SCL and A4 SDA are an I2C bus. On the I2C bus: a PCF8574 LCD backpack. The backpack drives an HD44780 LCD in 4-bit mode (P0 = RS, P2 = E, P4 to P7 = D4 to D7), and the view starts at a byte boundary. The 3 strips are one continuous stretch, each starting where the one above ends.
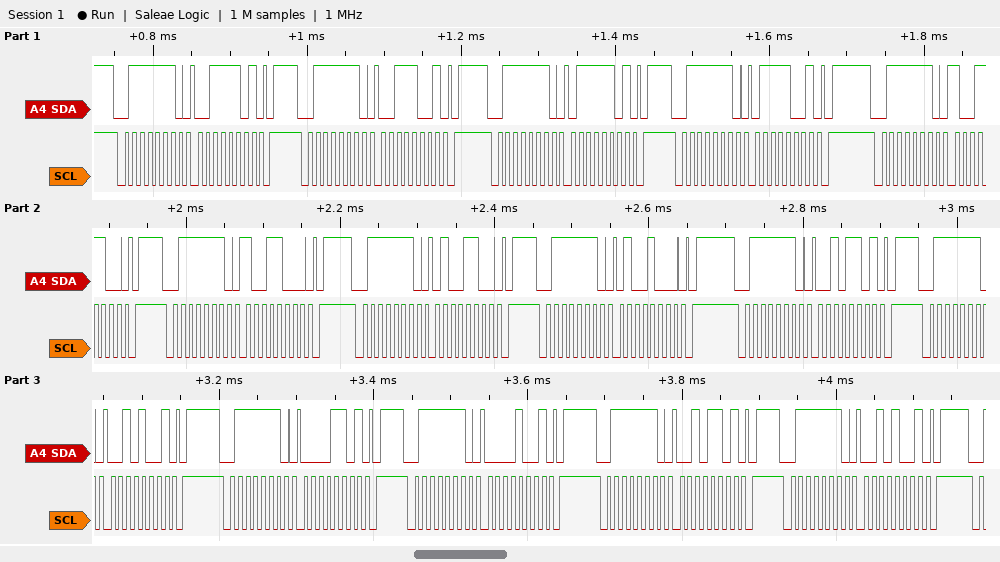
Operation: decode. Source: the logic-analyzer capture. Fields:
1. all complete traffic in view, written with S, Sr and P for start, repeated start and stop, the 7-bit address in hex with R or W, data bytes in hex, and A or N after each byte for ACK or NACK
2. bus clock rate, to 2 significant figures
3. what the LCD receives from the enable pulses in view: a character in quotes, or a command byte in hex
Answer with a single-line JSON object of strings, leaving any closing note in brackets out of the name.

{"all complete traffic in view, written with S, Sr and P for start, repeated start and stop, the 7-bit address in hex with R or W, data bytes in hex, and A or N after each byte for ACK or NACK": "S 3FW A 3D A P S 3FW A 39 A P S 3FW A 7D A P S 3FW A 79 A P S 3FW A 9C A P S 3FW A 98 A P S 3FW A 4C A P S 3FW A 48 A P S 3FW A 2D A P S 3FW A 29 A P S 3FW A 0D A P S 3FW A 09 A P S 3FW A 2D A P S 3FW A 29 A P", "bus clock rate, to 2 significant figures": "100 kHz", "what the LCD receives from the enable pulses in view: a character in quotes, or a command byte in hex": "'7' 0x94 ' '"}
